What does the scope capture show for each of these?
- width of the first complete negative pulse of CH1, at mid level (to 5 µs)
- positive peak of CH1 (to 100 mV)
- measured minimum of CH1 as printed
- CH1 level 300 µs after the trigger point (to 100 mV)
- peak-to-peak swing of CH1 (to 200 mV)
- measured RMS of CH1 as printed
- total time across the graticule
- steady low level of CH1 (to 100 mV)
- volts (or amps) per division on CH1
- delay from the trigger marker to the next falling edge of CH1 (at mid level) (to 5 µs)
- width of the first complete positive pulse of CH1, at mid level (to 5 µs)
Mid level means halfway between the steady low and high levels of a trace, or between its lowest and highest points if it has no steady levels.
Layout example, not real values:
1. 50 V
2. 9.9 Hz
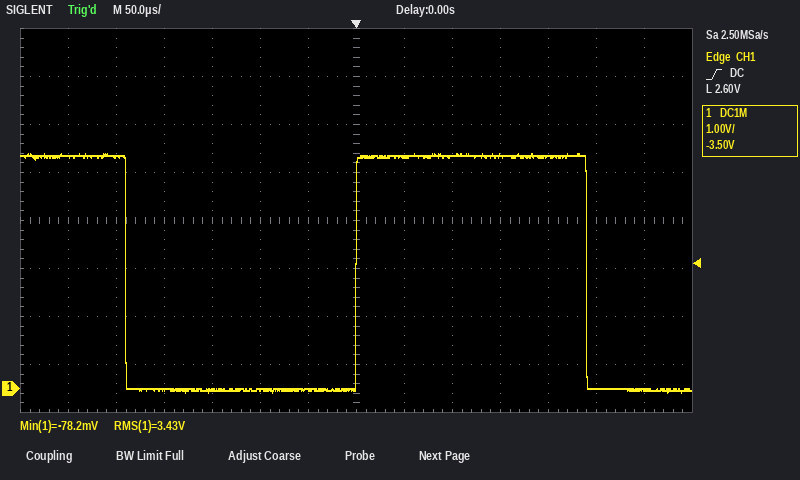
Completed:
1. 240 µs
2. 4.9 V
3. -78.2 mV
4. 0.0 V
5. 5.0 V
6. 3.43 V
7. 700 µs
8. 0.0 V
9. 1 V
10. 240 µs
11. 240 µs
